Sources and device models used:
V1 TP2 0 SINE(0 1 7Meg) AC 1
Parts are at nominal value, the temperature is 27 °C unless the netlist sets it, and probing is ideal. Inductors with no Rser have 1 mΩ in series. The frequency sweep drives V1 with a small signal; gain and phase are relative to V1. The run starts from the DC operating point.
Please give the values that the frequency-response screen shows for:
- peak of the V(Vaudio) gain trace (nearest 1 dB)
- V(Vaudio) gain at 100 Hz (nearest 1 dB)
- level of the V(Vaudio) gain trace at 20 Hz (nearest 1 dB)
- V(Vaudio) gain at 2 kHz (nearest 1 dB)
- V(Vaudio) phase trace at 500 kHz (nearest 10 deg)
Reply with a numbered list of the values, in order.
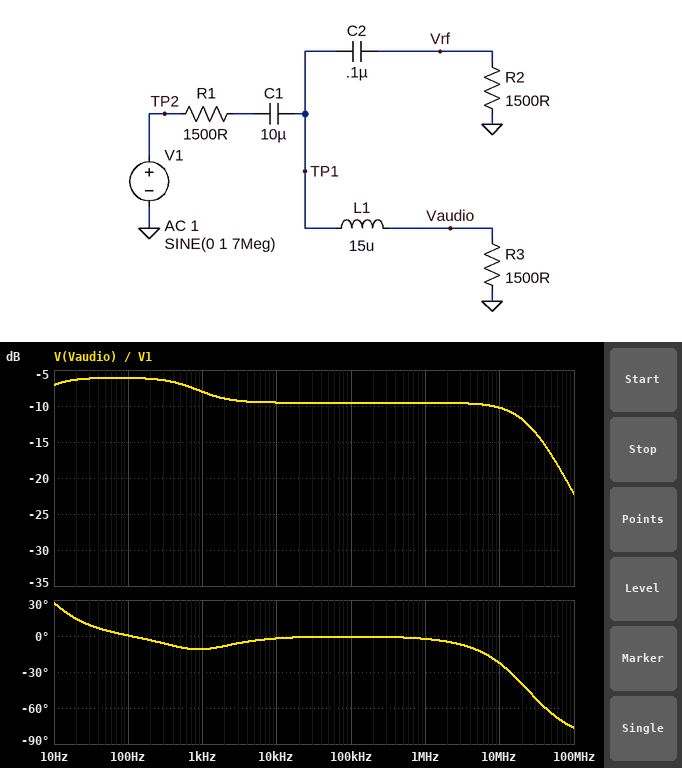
1. -6 dB
2. -6 dB
3. -6 dB
4. -9 dB
5. 0 deg
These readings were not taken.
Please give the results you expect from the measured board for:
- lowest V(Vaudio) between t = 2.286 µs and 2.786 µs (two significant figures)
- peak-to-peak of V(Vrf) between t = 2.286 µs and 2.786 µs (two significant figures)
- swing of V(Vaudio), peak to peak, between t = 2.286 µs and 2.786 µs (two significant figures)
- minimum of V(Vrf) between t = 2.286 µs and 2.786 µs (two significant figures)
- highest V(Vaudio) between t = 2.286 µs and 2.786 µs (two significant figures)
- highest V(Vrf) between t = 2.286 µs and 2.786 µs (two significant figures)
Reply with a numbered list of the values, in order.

1. -320 mV
2. 700 mV
3. 640 mV
4. -350 mV
5. 320 mV
6. 350 mV
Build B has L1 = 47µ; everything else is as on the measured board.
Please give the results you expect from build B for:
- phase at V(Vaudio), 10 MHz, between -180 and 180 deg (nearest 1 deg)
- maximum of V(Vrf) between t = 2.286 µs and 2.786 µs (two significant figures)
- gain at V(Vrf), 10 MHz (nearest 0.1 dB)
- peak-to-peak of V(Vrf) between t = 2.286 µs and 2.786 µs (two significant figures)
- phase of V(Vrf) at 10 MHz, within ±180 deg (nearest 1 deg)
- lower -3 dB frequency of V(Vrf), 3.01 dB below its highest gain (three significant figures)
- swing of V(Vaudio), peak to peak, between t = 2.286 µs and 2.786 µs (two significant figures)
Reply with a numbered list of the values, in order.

1. -53 deg
2. 420 mV
3. -7.0 dB
4. 840 mV
5. 10 deg
6. 2.54 MHz
7. 490 mV
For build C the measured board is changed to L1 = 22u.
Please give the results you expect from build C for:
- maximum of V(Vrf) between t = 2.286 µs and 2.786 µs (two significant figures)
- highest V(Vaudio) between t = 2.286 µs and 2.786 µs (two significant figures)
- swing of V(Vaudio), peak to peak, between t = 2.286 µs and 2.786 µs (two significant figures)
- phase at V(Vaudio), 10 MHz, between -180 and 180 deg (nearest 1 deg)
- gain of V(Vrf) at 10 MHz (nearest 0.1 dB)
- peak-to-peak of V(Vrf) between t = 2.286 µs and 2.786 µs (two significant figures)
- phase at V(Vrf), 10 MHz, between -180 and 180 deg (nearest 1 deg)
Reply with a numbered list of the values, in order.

1. 360 mV
2. 310 mV
3. 610 mV
4. -32 deg
5. -8.3 dB
6. 730 mV
7. 11 deg
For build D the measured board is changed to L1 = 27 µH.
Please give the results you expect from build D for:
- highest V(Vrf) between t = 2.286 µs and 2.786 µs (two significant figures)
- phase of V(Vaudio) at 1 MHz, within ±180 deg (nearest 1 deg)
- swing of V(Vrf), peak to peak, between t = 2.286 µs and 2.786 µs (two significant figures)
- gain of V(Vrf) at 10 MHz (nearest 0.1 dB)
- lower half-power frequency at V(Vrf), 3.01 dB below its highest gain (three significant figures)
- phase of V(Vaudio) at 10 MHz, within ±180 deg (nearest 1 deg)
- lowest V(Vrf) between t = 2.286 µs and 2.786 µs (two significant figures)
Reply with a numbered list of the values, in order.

1. 380 mV
2. -4 deg
3. 750 mV
4. -7.9 dB
5. 4.42 MHz
6. -37 deg
7. -380 mV
